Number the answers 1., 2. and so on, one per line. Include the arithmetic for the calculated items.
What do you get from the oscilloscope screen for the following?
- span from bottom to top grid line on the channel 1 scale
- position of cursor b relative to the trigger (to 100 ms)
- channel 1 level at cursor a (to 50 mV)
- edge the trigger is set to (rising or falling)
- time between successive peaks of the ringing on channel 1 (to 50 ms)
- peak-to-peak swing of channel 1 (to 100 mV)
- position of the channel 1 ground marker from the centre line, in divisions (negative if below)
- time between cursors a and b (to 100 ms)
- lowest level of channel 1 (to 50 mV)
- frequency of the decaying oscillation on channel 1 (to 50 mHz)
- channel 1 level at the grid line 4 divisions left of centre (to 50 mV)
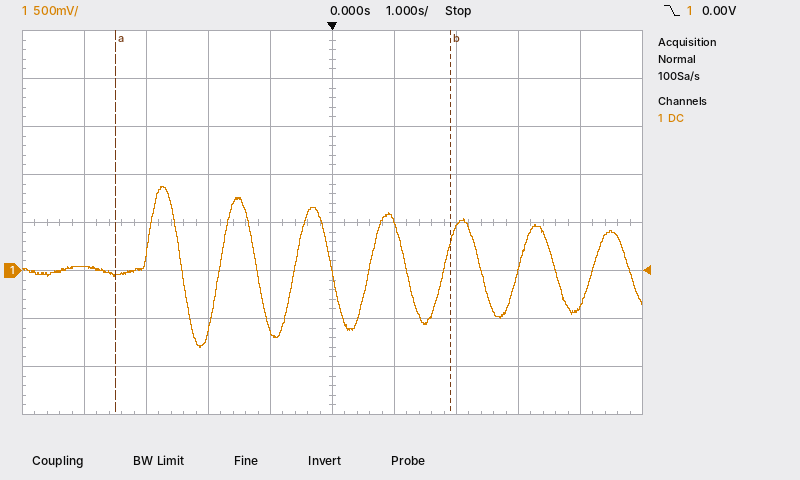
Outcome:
1. 4 V
2. +1.9 s
3. -50 mV
4. falling
5. 1.20 s
6. 1.70 V
7. -1.0 div
8. 5.4 s
9. -800 mV
10. 1 / 1.20 s ≈ 833 mHz, so 850 mHz to the nearest 50 mHz
11. 50 mV
